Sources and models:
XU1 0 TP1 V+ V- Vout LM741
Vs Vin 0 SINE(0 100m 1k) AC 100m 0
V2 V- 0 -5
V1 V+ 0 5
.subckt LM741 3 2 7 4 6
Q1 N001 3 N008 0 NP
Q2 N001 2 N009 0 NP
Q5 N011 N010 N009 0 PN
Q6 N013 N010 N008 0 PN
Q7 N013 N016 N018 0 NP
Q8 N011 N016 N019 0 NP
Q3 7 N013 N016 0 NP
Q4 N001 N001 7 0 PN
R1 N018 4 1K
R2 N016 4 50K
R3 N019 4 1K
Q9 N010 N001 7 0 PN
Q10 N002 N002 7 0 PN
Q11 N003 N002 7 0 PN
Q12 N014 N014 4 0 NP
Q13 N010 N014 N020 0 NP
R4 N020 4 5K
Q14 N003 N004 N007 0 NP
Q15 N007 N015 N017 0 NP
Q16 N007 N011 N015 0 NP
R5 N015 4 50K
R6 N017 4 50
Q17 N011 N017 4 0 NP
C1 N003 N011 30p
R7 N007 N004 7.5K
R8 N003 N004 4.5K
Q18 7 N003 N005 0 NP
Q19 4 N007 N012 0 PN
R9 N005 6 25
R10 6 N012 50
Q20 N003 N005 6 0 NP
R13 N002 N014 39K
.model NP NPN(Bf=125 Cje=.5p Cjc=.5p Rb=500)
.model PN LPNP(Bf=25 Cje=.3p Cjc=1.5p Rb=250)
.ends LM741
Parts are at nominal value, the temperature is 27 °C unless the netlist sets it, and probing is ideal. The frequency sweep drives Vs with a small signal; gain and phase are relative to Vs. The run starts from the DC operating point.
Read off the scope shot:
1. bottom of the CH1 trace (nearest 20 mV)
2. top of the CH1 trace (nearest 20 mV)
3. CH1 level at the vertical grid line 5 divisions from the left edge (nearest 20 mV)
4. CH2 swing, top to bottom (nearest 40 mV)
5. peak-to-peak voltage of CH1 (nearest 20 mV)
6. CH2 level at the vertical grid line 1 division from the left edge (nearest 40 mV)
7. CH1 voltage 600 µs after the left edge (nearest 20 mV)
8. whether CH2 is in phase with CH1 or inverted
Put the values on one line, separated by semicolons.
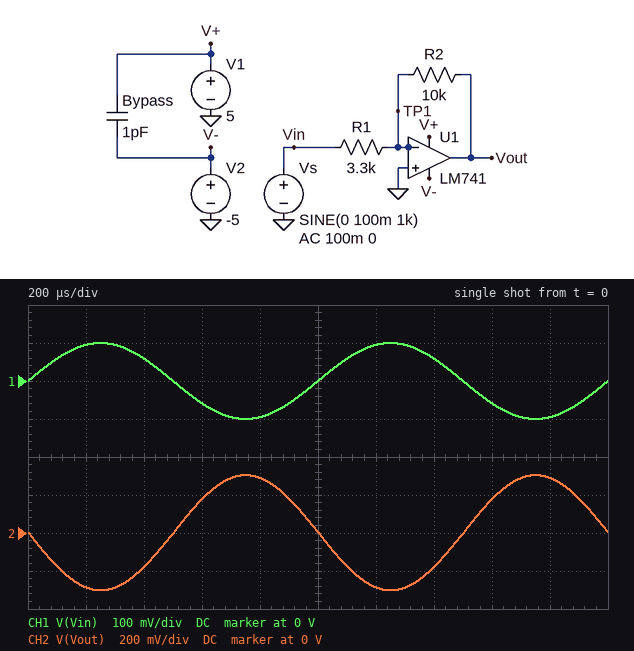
-100 mV; 100 mV; 0 V; 600 mV; 200 mV; -280 mV; -60 mV; inverted
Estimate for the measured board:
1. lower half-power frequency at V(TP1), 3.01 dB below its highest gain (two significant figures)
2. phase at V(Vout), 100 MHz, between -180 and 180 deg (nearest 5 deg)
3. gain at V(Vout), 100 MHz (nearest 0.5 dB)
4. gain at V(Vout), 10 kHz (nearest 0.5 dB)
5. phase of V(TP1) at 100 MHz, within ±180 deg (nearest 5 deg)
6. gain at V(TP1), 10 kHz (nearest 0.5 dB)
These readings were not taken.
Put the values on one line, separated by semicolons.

57 kHz; -85 deg; -24.0 dB; 9.5 dB; -30 deg; -16.0 dB
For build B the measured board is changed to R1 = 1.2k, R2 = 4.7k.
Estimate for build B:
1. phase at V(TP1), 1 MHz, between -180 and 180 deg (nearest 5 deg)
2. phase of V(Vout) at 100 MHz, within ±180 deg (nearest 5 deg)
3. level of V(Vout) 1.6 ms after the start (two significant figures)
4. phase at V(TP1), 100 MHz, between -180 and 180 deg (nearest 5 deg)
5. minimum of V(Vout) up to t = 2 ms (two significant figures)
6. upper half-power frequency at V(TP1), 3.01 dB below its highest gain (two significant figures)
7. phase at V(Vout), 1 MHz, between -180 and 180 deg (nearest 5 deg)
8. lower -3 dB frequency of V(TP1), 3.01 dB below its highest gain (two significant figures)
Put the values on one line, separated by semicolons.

0 deg; -70 deg; 230 mV; -15 deg; -390 mV; 130 MHz; 5 deg; 26 kHz
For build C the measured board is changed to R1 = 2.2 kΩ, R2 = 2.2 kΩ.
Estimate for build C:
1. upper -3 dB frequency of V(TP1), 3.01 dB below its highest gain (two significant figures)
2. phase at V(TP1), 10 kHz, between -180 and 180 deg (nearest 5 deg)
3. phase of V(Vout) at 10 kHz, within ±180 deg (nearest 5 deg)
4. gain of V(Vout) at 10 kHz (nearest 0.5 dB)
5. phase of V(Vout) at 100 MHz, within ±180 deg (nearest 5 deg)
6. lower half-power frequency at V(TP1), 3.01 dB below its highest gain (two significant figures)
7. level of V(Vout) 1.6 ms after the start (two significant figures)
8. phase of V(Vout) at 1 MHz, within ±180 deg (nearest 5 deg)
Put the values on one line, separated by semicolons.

30 MHz; 80 deg; 160 deg; 0 dB; -70 deg; 49 kHz; 59 mV; 5 deg
